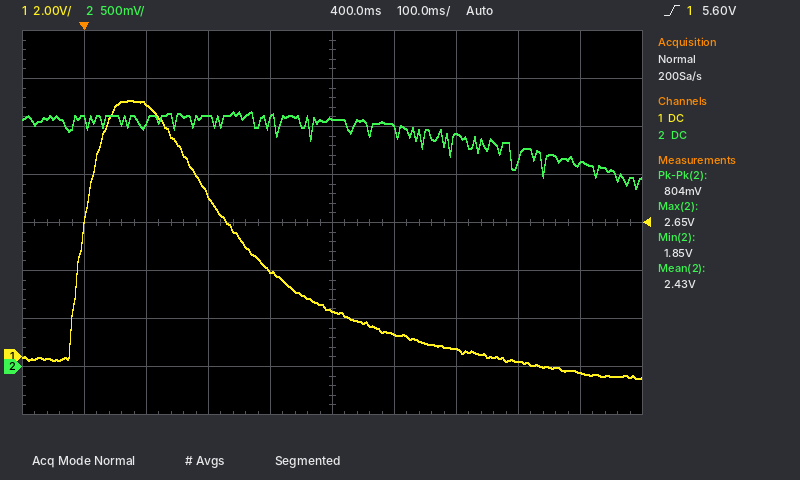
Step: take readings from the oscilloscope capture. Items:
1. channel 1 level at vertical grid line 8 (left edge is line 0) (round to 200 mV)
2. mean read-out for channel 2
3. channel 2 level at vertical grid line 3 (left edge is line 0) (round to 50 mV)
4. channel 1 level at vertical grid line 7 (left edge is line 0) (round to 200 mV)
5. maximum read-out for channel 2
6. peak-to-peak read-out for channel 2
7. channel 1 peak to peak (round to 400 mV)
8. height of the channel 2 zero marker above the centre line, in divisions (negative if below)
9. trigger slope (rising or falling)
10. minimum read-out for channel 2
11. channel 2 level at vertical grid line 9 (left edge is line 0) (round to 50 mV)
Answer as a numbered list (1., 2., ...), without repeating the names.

1. -200 mV
2. 2.43 V
3. 2.60 V
4. 400 mV
5. 2.65 V
6. 804 mV
7. 11.6 V
8. -3.0 div
9. rising
10. 1.85 V
11. 2.10 V
